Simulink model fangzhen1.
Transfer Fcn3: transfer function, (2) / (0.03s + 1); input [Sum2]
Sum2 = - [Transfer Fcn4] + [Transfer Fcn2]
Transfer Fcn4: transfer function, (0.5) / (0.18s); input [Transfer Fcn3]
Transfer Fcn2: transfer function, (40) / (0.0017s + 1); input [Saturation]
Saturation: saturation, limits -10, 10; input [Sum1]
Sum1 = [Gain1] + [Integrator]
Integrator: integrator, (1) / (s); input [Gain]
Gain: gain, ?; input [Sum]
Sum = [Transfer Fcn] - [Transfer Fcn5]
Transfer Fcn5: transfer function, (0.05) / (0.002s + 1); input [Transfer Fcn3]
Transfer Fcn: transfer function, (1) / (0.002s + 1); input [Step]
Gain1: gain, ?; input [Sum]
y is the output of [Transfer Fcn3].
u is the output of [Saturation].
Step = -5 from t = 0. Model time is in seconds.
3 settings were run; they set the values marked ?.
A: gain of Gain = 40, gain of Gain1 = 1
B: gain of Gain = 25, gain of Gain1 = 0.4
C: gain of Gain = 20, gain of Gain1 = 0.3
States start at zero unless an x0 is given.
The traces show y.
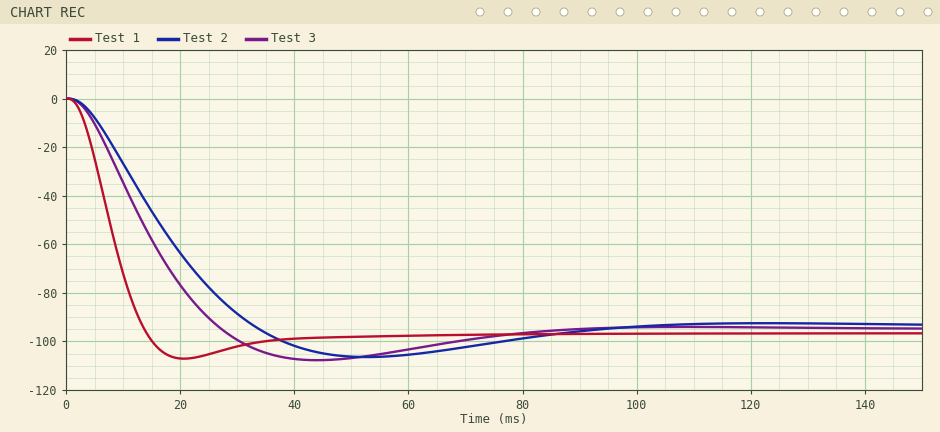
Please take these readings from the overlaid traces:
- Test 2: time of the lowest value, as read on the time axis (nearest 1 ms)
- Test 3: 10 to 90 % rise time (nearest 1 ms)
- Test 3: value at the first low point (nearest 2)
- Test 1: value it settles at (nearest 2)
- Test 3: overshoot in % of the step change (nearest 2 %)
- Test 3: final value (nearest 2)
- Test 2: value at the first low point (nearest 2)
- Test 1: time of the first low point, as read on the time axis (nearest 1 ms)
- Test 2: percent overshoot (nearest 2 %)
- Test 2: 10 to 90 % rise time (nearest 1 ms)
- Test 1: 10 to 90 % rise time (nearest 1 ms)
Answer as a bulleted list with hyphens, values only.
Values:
- 53 ms
- 18 ms
- -108
- -96
- 14 %
- -94
- -106
- 21 ms
- 14 %
- 22 ms
- 9 ms
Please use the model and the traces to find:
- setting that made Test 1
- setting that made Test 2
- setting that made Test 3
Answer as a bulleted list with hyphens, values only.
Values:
- A
- C
- B
